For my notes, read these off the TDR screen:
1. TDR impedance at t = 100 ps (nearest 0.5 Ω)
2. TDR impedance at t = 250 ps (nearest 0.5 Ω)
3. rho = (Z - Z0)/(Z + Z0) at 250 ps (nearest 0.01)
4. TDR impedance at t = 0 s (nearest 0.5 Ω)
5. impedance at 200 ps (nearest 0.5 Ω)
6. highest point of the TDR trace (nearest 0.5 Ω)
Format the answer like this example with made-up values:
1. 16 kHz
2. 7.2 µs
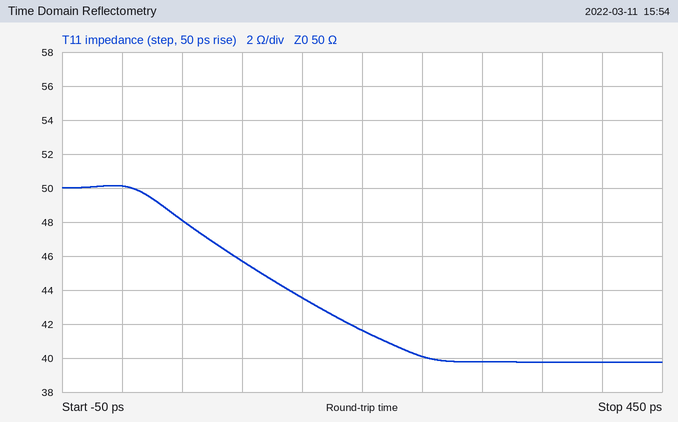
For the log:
1. 45.5 Ω
2. 40.0 Ω
3. -0.11
4. 50.0 Ω
5. 41.5 Ω
6. 50.0 Ω
